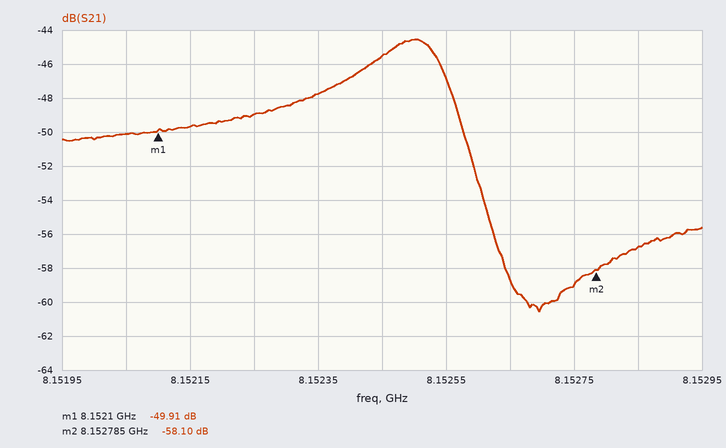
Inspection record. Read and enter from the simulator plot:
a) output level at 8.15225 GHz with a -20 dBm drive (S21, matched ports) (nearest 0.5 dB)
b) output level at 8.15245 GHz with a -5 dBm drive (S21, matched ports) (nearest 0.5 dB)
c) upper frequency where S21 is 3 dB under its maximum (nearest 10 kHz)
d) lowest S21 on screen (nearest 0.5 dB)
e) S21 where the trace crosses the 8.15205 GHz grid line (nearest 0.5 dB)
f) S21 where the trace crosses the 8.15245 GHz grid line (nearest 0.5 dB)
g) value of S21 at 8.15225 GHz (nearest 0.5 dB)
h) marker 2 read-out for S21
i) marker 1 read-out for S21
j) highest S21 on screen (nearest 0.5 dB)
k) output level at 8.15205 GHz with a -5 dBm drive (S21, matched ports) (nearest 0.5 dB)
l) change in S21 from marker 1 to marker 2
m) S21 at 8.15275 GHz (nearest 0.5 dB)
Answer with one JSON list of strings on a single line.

["-69.0 dBm", "-50.5 dBm", "8.15256 GHz", "-60.5 dB", "-50.0 dB", "-45.5 dB", "-49.0 dB", "-58.10 dB", "-49.91 dB", "-44.5 dB", "-55.0 dBm", "-8.19 dB", "-59.0 dB"]
